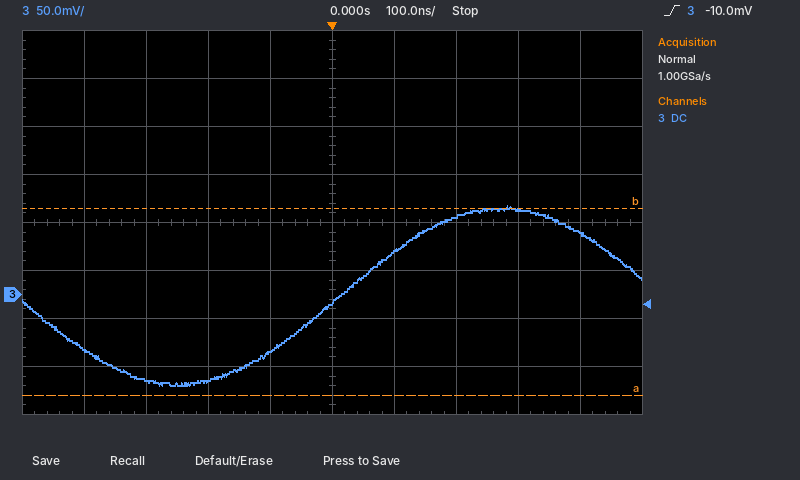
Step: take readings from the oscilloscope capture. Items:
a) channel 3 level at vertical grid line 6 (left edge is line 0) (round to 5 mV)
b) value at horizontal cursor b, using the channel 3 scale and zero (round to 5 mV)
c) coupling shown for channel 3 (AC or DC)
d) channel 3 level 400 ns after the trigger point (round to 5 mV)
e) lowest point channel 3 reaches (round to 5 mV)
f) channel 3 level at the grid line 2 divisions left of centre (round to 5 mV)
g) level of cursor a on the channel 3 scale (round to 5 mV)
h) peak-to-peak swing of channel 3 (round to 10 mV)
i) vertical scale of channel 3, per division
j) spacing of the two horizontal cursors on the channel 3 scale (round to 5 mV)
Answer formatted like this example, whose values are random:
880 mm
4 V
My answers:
45 mV
90 mV
DC
65 mV
-95 mV
-90 mV
-105 mV
190 mV
50 mV
195 mV
